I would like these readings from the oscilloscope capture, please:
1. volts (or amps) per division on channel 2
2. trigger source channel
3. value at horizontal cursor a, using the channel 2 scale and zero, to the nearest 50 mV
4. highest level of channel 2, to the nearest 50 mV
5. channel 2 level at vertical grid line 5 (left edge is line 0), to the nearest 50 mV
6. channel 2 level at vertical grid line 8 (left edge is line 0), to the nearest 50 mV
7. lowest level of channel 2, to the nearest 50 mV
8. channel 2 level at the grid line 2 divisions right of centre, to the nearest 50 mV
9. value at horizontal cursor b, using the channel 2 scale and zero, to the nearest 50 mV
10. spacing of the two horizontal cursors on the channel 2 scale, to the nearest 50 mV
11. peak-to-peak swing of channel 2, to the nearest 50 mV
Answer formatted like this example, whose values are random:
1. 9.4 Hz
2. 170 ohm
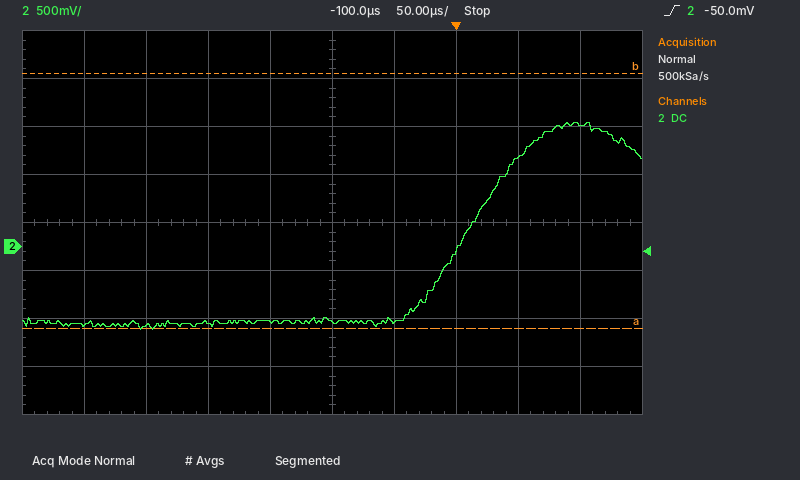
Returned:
1. 500 mV
2. channel 2
3. -850 mV
4. 1.30 V
5. -800 mV
6. 950 mV
7. -850 mV
8. -50 mV
9. 1.80 V
10. 2.65 V
11. 2.15 V
